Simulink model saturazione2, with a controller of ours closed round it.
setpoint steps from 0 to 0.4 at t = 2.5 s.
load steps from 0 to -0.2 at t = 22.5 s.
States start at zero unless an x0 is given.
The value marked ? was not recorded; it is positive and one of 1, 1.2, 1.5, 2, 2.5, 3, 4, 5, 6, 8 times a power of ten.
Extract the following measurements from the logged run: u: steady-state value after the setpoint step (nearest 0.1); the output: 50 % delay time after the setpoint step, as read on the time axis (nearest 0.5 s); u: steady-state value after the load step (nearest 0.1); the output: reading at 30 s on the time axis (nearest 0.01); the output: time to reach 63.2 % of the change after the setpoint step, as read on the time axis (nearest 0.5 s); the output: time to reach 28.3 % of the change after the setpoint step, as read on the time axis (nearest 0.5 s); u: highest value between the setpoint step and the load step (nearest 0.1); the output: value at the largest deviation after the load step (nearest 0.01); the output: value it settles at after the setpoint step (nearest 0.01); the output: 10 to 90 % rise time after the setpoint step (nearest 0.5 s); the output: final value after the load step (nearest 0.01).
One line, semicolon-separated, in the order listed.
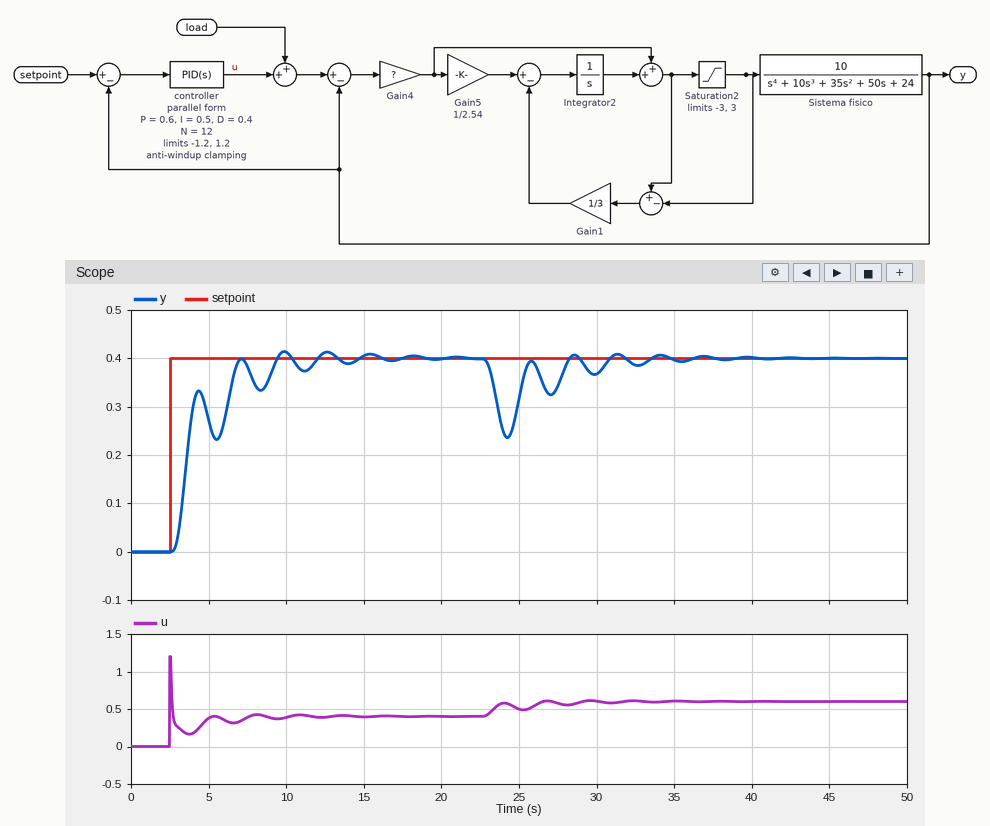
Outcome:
0.4; 3.5 s; 0.6; 0.37; 4.0 s; 3.5 s; 1.2; 0.24; 0.40; 3.5 s; 0.40
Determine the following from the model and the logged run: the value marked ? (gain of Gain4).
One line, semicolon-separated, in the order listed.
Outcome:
6
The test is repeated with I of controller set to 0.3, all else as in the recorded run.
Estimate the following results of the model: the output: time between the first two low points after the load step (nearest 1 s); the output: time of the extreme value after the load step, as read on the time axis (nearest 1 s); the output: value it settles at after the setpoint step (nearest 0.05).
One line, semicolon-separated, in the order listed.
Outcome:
3 s; 24 s; 0.40
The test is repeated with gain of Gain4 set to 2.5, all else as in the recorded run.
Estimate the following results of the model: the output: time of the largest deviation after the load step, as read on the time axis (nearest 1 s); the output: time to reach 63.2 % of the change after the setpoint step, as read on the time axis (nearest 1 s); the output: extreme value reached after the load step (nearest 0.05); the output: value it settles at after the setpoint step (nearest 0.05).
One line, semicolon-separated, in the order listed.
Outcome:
25 s; 5 s; 0.30; 0.40
